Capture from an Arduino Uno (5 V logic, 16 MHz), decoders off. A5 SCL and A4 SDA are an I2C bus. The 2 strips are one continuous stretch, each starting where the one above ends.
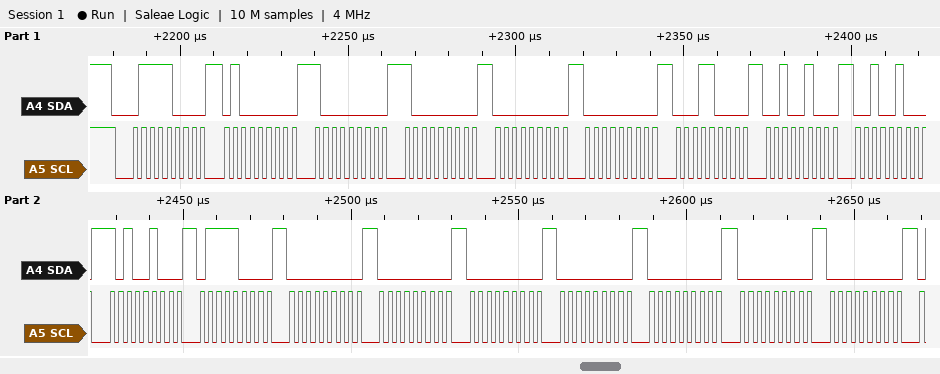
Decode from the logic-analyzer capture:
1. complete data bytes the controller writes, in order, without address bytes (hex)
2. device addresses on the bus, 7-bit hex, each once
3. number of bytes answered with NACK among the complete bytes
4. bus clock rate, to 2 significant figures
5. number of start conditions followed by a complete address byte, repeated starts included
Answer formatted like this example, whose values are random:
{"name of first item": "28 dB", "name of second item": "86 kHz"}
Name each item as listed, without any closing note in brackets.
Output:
{"complete data bytes the controller writes, in order, without address bytes": "40 80 80 00 00 18 24 24 A4 78 00 00 00 00 00 00 00", "device addresses on the bus, 7-bit hex, each once": "0x3C", "number of bytes answered with NACK among the complete bytes": "0", "bus clock rate, to 2 significant figures": "400 kHz", "number of start conditions followed by a complete address byte, repeated starts included": "1"}
